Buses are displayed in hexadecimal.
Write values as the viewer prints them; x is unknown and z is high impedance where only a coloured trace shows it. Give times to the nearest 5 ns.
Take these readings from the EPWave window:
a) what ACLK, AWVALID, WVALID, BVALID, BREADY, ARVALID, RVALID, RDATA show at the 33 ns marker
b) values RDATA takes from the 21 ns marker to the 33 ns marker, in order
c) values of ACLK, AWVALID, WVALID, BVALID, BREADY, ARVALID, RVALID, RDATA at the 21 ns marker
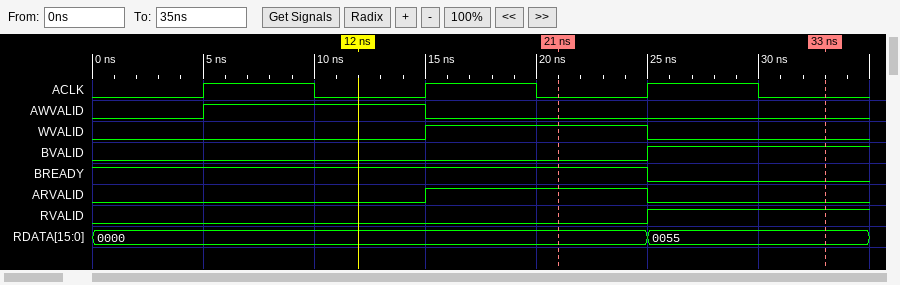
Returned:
ACLK=0, AWVALID=0, WVALID=0, BVALID=1, BREADY=0, ARVALID=0, RVALID=1, RDATA=0055
0000, 0055
ACLK=0, AWVALID=0, WVALID=1, BVALID=0, BREADY=1, ARVALID=1, RVALID=0, RDATA=0000
